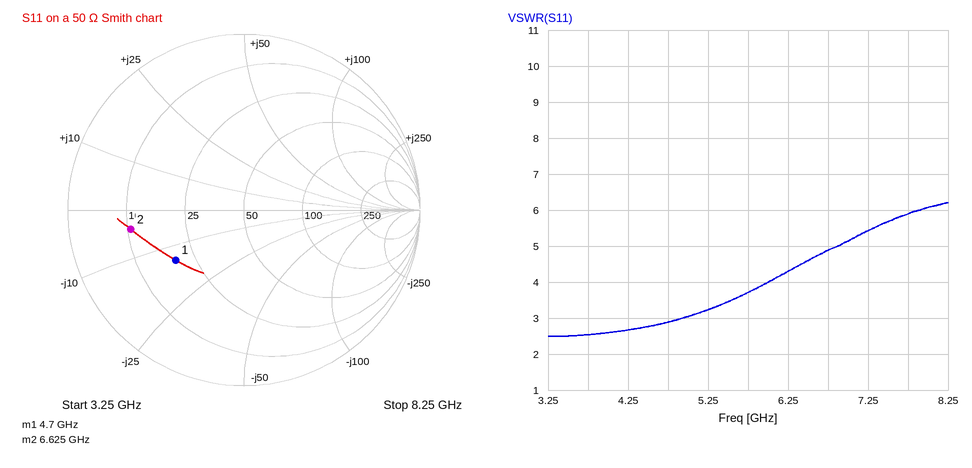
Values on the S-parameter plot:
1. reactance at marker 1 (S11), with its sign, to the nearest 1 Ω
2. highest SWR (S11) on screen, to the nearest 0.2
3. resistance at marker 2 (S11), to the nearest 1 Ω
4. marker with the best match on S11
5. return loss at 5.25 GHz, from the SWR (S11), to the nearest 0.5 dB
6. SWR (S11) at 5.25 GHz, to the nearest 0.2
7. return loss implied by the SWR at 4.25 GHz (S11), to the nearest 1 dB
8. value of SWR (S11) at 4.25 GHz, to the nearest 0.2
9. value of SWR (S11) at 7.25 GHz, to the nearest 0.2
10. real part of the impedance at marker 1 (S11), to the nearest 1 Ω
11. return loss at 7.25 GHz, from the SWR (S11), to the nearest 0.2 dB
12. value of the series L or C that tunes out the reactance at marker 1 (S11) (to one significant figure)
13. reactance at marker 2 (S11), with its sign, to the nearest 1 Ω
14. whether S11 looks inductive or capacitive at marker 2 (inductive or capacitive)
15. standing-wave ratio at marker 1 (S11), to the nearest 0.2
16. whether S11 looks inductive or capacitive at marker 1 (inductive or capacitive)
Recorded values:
-14 Ω
6.2
11 Ω
marker 1
5.5 dB
3.2
7 dB
2.6
5.4
19 Ω
3.2 dB
500 pH
-4 Ω
capacitive
2.8
capacitive
